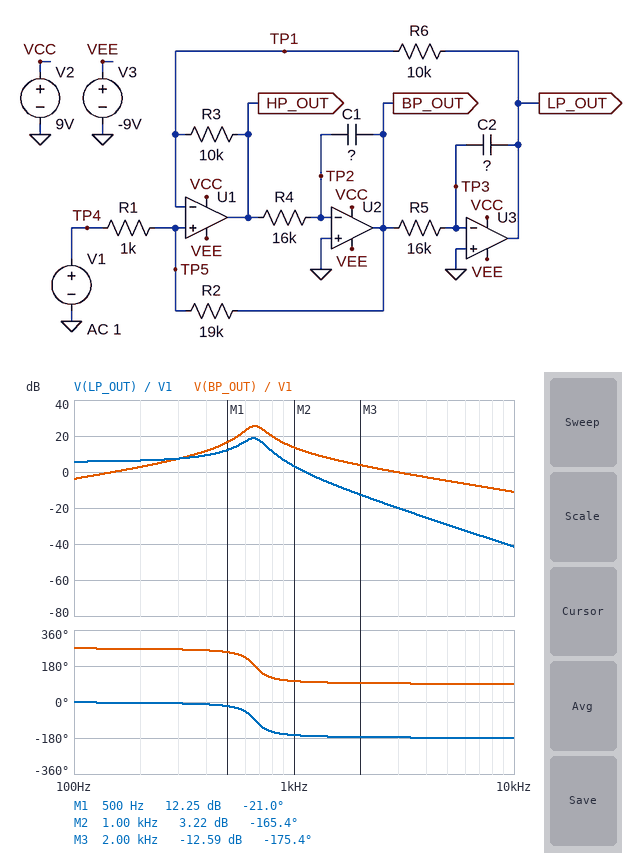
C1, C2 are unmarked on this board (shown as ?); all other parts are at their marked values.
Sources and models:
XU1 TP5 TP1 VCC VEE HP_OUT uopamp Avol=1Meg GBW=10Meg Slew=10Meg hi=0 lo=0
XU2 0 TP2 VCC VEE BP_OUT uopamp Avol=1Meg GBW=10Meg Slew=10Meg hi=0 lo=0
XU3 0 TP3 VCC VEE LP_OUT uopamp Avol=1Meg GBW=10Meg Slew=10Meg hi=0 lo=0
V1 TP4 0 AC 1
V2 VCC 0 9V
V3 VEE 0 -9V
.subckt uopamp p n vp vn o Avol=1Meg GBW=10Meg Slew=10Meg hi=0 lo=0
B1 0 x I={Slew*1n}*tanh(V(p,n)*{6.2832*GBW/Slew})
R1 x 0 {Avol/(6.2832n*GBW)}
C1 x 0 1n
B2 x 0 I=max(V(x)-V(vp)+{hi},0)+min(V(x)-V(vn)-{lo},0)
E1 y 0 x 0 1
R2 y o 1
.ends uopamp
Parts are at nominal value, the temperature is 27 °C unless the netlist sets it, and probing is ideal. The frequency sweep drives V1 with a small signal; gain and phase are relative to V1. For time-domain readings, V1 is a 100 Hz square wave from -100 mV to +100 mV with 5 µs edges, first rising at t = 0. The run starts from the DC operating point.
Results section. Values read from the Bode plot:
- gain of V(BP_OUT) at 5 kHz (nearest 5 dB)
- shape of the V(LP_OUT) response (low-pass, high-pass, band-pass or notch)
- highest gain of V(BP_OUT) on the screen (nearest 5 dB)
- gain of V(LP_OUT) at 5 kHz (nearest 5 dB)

-5 dB
low-pass
25 dB
-30 dB
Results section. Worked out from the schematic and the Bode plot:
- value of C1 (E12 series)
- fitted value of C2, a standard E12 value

6.8 nF
33 nF
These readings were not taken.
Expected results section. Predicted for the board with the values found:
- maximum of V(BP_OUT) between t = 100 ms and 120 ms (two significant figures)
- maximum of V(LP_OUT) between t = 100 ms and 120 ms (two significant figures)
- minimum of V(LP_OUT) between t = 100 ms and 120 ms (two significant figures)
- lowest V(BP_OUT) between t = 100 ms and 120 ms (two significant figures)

720 mV
460 mV
-460 mV
-720 mV
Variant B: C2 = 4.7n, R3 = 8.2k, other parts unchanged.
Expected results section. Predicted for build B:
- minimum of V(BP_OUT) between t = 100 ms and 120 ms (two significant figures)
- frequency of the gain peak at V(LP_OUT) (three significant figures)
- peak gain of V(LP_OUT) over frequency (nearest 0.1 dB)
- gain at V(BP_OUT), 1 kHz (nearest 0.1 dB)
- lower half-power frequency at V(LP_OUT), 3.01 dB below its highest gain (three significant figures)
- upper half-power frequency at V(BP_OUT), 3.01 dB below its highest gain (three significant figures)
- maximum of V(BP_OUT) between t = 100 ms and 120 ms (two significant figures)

-270 mV
1.59 kHz
28.1 dB
4.3 dB
1.52 kHz
1.66 kHz
270 mV
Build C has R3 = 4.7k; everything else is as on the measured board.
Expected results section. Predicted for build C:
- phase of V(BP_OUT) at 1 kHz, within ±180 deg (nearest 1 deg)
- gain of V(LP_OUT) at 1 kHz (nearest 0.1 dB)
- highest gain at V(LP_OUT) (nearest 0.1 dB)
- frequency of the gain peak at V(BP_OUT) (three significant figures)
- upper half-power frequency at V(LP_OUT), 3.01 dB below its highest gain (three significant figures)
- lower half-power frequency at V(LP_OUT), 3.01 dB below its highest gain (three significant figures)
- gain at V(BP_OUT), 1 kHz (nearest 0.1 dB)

98 deg
-2.3 dB
22.1 dB
455 Hz
500 Hz
391 Hz
8.1 dB
